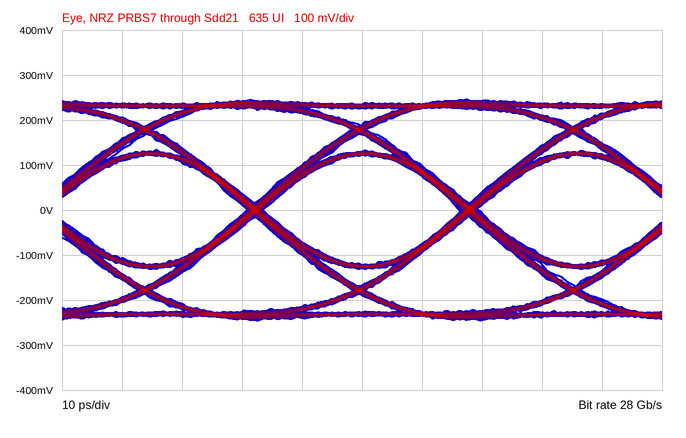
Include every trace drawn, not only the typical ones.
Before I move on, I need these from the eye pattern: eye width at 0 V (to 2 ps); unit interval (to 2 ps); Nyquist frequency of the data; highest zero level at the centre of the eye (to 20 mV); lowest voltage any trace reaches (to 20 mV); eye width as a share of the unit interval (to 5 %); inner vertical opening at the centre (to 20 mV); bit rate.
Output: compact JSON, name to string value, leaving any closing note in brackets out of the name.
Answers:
{"eye width at 0 V": "32 ps", "unit interval": "36 ps", "Nyquist frequency of the data": "14 GHz", "highest zero level at the centre of the eye": "-120 mV", "lowest voltage any trace reaches": "-240 mV", "eye width as a share of the unit interval": "90 %", "inner vertical opening at the centre": "240 mV", "bit rate": "28 Gb/s"}
